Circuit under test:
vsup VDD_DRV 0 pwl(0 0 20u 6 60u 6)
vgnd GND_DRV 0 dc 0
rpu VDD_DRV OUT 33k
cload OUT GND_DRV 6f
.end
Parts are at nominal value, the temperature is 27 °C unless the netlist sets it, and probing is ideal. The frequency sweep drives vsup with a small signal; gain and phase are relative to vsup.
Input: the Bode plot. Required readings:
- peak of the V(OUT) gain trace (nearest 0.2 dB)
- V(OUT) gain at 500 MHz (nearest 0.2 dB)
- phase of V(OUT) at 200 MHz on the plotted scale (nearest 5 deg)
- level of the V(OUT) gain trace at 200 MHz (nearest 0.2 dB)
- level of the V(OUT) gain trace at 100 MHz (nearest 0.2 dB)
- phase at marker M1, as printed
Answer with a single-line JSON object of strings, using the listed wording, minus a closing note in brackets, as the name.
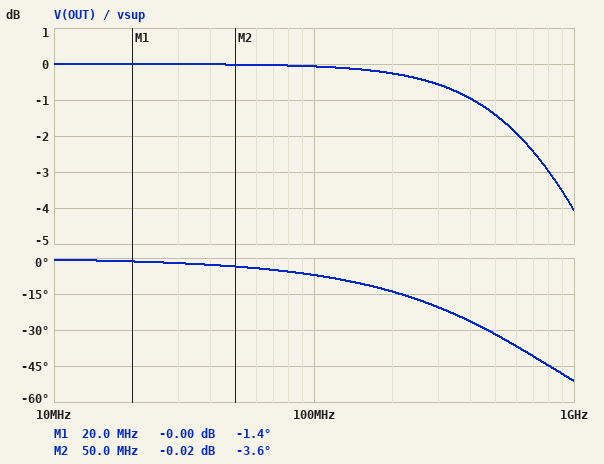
{"peak of the V(OUT) gain trace": "0 dB", "V(OUT) gain at 500 MHz": "-1.4 dB", "phase of V(OUT) at 200 MHz on the plotted scale": "-15 deg", "level of the V(OUT) gain trace at 200 MHz": "-0.2 dB", "level of the V(OUT) gain trace at 100 MHz": "0 dB", "phase at marker M1, as printed": "-1.4 deg"}
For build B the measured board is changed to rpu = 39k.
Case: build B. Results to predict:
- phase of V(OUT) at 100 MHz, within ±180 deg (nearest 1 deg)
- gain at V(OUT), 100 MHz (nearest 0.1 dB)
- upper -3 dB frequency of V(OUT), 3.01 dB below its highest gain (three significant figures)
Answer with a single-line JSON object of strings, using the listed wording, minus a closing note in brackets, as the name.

{"phase of V(OUT) at 100 MHz, within ±180 deg": "-8 deg", "gain at V(OUT), 100 MHz": "-0.1 dB", "upper -3 dB frequency of V(OUT), 3.01 dB below its highest gain": "680 MHz"}
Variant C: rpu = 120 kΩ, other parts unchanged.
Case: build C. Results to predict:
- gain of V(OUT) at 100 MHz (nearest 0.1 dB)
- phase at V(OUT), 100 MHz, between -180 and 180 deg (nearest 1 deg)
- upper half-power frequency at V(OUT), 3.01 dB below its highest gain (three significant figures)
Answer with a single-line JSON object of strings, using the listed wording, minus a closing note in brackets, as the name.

{"gain of V(OUT) at 100 MHz": "-0.8 dB", "phase at V(OUT), 100 MHz, between -180 and 180 deg": "-24 deg", "upper half-power frequency at V(OUT), 3.01 dB below its highest gain": "221 MHz"}
